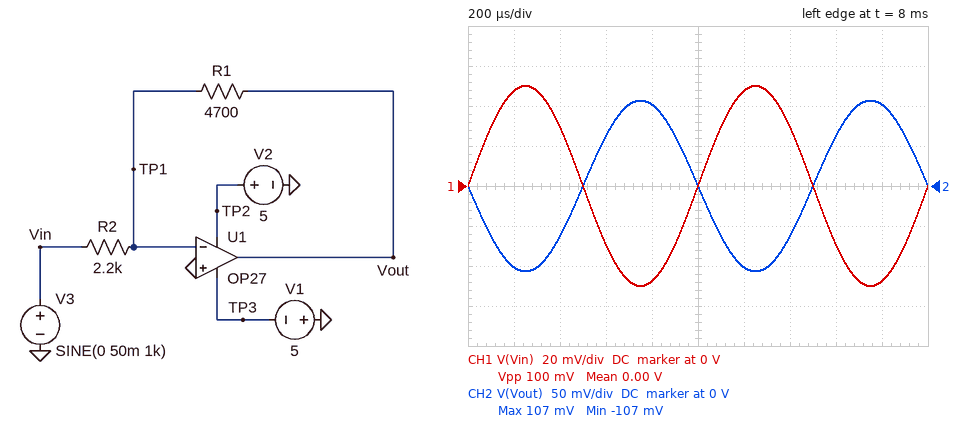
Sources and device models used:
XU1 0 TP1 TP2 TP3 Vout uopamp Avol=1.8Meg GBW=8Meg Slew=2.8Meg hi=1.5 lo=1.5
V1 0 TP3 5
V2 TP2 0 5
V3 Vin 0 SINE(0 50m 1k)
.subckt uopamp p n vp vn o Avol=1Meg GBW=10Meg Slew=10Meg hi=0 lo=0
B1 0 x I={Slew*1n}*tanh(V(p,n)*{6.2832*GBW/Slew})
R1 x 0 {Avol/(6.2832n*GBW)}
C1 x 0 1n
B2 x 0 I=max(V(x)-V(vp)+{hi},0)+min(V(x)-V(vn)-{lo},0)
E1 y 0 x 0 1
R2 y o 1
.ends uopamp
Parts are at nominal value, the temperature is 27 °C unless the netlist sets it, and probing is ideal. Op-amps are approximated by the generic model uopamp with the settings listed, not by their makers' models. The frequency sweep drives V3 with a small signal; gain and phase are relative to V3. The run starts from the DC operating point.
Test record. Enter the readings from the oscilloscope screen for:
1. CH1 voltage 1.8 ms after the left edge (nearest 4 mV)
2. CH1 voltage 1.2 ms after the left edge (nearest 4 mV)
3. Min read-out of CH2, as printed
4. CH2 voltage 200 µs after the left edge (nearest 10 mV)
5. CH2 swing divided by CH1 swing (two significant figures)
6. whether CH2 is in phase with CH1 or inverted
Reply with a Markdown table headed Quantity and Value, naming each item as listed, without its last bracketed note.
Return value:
| Quantity | Value |
|---|---|
| CH1 voltage 1.8 ms after the left edge | -48 mV |
| CH1 voltage 1.2 ms after the left edge | 48 mV |
| Min read-out of CH2, as printed | -107 mV |
| CH2 voltage 200 µs after the left edge | -100 mV |
| CH2 swing divided by CH1 swing | 2.1 |
| whether CH2 is in phase with CH1 or inverted | inverted |
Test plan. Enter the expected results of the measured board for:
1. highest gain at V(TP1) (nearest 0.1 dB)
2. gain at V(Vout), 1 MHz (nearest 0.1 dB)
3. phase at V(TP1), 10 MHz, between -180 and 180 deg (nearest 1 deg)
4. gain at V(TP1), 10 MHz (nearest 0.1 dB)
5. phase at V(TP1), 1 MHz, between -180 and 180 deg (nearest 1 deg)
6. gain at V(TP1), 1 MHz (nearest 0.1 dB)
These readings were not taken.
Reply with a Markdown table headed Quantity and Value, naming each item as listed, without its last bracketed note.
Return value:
| Quantity | Value |
|---|---|
| highest gain at V(TP1) | -3.3 dB |
| gain at V(Vout), 1 MHz | 6.0 dB |
| phase at V(TP1), 10 MHz, between -180 and 180 deg | 14 deg |
| gain at V(TP1), 10 MHz | -3.6 dB |
| phase at V(TP1), 1 MHz, between -180 and 180 deg | 69 deg |
| gain at V(TP1), 1 MHz | -12.1 dB |
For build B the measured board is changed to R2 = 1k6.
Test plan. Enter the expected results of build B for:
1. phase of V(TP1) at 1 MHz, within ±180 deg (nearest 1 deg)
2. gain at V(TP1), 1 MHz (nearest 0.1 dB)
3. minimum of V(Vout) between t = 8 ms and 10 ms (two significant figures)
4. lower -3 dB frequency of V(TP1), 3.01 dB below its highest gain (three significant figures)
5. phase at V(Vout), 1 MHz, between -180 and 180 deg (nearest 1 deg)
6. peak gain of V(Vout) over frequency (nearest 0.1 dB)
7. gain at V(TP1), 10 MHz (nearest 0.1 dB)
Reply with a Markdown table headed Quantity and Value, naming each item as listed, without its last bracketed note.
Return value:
| Quantity | Value |
|---|---|
| phase of V(TP1) at 1 MHz, within ±180 deg | 64 deg |
| gain at V(TP1), 1 MHz | -9.6 dB |
| minimum of V(Vout) between t = 8 ms and 10 ms | -150 mV |
| lower -3 dB frequency of V(TP1), 3.01 dB below its highest gain | 2.03 MHz |
| phase at V(Vout), 1 MHz, between -180 and 180 deg | 154 deg |
| peak gain of V(Vout) over frequency | 9.4 dB |
| gain at V(TP1), 10 MHz | -2.7 dB |
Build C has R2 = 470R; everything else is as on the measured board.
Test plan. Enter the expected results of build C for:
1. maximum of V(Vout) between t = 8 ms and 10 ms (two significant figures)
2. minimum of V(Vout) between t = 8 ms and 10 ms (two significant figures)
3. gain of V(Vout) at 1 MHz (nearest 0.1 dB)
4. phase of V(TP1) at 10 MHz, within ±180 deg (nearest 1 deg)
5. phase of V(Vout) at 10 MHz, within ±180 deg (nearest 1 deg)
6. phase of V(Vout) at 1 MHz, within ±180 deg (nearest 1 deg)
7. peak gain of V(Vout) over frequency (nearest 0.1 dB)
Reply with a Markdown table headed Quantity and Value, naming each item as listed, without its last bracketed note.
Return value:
| Quantity | Value |
|---|---|
| maximum of V(Vout) between t = 8 ms and 10 ms | 500 mV |
| minimum of V(Vout) between t = 8 ms and 10 ms | -500 mV |
| gain of V(Vout) at 1 MHz | 15.4 dB |
| phase of V(TP1) at 10 MHz, within ±180 deg | 4 deg |
| phase of V(Vout) at 10 MHz, within ±180 deg | 94 deg |
| phase of V(Vout) at 1 MHz, within ±180 deg | 126 deg |
| peak gain of V(Vout) over frequency | 20.0 dB |
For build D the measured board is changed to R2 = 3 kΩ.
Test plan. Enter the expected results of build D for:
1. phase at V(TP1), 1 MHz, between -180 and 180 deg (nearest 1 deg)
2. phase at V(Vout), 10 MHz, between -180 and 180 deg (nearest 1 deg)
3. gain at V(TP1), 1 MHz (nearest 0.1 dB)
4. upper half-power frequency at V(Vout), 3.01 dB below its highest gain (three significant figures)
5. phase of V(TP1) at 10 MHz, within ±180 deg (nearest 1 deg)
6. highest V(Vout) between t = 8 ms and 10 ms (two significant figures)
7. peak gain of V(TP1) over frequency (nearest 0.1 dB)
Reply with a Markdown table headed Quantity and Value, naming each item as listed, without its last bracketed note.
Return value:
| Quantity | Value |
|---|---|
| phase at V(TP1), 1 MHz, between -180 and 180 deg | 72 deg |
| phase at V(Vout), 10 MHz, between -180 and 180 deg | 107 deg |
| gain at V(TP1), 1 MHz | -14.6 dB |
| upper half-power frequency at V(Vout), 3.01 dB below its highest gain | 3.12 MHz |
| phase of V(TP1) at 10 MHz, within ±180 deg | 17 deg |
| highest V(Vout) between t = 8 ms and 10 ms | 78 mV |
| peak gain of V(TP1) over frequency | -4.3 dB |
